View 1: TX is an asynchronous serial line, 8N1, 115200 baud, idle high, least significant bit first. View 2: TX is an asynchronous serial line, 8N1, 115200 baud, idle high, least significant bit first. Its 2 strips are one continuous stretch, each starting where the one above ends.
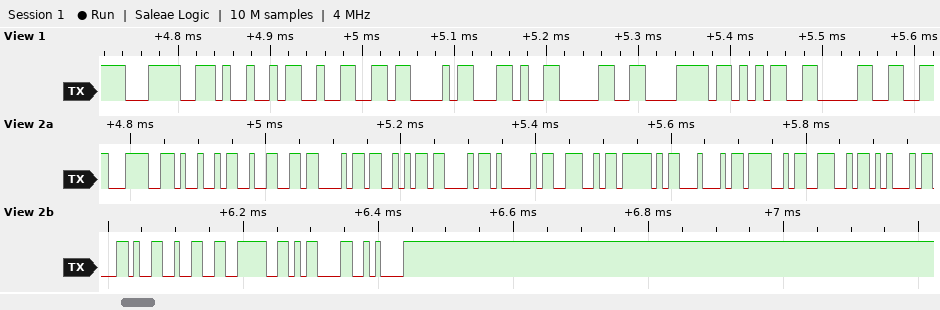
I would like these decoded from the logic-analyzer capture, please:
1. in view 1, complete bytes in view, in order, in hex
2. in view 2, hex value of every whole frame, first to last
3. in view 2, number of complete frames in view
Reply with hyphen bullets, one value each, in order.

- 3C 49 32 43 2C 30 78 35 30
- 3C 49 32 43 53 43 41 4E 5F 44 4F 4E 45 2C 32 3E 0D 0A
- 18
